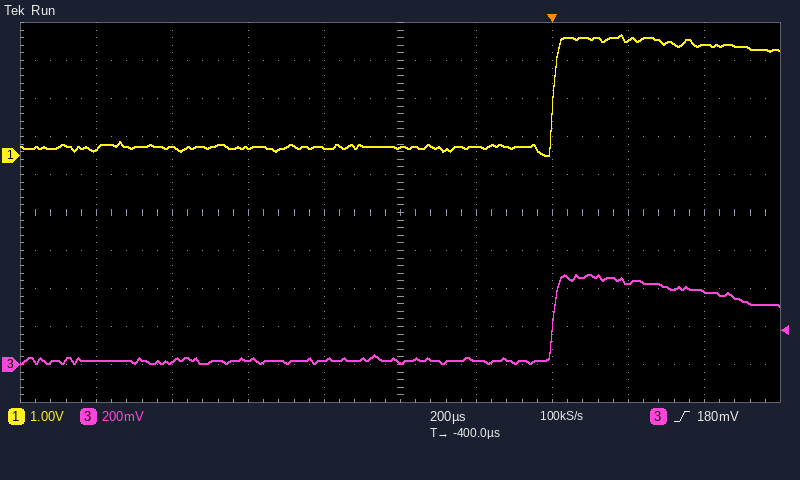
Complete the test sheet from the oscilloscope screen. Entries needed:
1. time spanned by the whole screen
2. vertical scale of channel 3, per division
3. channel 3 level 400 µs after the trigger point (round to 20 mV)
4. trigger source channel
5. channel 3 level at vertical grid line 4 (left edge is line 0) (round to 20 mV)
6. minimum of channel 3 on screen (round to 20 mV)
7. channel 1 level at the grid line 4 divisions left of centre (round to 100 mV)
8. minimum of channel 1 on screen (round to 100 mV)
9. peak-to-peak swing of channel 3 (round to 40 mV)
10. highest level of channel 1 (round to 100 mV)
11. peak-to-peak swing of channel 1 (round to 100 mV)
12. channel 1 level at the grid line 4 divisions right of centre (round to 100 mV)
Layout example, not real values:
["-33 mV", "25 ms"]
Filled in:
["2 ms", "200 mV", "380 mV", "channel 3", "20 mV", "0 mV", "200 mV", "0.0 V", "480 mV", "3.2 V", "3.2 V", "2.9 V"]
